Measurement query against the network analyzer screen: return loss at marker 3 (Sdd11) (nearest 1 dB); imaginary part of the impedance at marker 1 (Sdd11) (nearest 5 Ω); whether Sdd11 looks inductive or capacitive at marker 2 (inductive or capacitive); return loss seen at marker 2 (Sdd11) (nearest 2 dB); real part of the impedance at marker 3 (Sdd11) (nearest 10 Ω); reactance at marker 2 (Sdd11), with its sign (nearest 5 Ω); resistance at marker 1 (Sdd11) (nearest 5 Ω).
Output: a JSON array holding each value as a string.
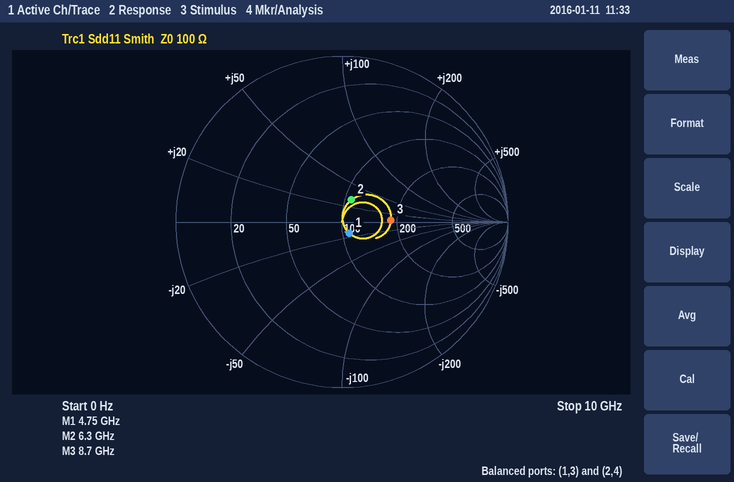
["11 dB", "-15 Ω", "inductive", "16 dB", "180 Ω", "+30 Ω", "110 Ω"]
